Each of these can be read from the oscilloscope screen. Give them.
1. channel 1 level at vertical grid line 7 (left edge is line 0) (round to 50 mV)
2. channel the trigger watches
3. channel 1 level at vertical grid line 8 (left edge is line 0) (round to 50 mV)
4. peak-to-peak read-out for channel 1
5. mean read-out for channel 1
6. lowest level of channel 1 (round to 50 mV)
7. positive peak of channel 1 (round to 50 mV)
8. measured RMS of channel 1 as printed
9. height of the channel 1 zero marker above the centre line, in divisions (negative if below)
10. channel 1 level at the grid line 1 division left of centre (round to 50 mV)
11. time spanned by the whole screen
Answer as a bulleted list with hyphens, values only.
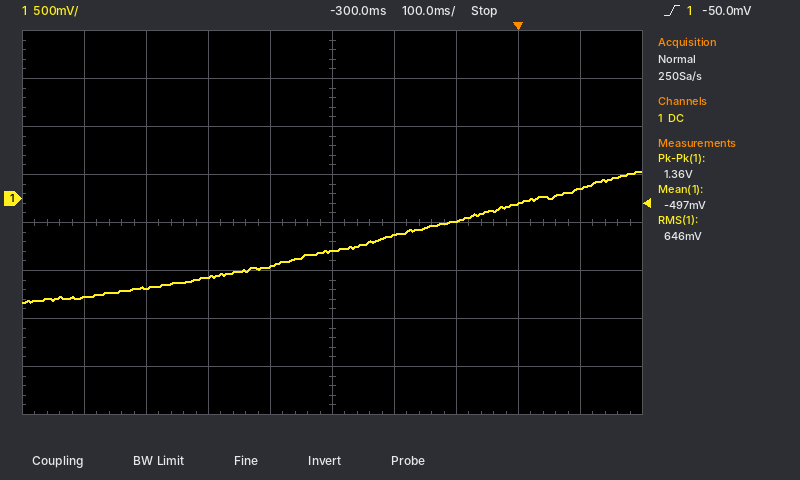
- -250 mV
- channel 1
- -50 mV
- 1.36 V
- -497 mV
- -1.10 V
- 300 mV
- 646 mV
- +0.5 div
- -700 mV
- 1 s
